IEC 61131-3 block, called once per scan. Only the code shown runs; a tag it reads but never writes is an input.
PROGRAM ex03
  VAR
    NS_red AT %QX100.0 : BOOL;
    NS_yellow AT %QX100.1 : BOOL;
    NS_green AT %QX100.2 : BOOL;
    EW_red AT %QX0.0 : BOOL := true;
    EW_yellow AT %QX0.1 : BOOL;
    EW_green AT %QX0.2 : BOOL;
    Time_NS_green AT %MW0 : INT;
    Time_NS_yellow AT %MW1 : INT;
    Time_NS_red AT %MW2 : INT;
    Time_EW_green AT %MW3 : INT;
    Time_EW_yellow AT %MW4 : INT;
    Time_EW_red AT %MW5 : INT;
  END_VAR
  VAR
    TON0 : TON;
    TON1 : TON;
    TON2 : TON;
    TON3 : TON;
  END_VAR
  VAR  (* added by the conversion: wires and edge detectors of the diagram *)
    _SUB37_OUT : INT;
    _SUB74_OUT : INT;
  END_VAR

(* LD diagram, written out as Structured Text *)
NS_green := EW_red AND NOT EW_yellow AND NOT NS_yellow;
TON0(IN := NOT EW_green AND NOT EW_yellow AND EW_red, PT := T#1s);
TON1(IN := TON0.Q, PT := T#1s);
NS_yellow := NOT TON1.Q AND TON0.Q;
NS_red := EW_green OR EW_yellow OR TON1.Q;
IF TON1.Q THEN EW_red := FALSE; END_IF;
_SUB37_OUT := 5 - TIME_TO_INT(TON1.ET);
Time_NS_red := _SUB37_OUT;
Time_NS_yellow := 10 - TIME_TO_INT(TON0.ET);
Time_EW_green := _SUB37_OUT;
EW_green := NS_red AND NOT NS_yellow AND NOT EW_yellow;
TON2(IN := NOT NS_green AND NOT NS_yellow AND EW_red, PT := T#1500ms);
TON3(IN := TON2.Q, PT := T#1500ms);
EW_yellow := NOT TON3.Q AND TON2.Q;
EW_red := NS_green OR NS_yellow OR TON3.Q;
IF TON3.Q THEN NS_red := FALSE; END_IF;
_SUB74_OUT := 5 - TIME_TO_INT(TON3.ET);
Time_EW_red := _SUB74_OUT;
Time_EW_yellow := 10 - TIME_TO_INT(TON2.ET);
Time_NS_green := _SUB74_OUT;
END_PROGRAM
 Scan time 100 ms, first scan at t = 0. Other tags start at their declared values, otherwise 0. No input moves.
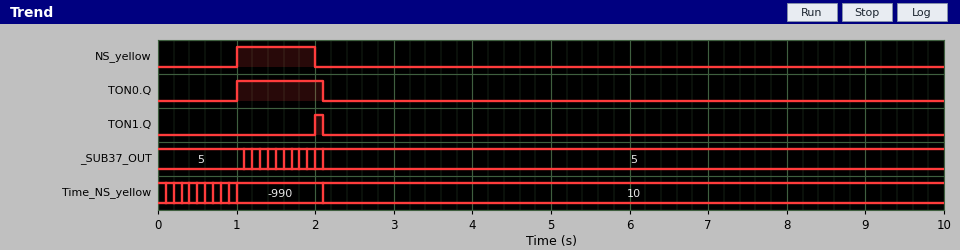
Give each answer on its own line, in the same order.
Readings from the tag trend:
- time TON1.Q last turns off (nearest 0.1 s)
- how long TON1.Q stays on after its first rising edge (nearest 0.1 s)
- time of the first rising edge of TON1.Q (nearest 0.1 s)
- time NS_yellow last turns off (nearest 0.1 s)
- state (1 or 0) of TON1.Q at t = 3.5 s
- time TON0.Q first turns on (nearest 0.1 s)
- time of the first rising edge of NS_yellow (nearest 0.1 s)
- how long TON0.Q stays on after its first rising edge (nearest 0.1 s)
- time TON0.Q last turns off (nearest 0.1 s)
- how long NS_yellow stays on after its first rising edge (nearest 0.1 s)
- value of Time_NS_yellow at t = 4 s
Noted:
2.1 s
0.1 s
2.0 s
2.0 s
0
1.0 s
1.0 s
1.1 s
2.1 s
1.0 s
10
